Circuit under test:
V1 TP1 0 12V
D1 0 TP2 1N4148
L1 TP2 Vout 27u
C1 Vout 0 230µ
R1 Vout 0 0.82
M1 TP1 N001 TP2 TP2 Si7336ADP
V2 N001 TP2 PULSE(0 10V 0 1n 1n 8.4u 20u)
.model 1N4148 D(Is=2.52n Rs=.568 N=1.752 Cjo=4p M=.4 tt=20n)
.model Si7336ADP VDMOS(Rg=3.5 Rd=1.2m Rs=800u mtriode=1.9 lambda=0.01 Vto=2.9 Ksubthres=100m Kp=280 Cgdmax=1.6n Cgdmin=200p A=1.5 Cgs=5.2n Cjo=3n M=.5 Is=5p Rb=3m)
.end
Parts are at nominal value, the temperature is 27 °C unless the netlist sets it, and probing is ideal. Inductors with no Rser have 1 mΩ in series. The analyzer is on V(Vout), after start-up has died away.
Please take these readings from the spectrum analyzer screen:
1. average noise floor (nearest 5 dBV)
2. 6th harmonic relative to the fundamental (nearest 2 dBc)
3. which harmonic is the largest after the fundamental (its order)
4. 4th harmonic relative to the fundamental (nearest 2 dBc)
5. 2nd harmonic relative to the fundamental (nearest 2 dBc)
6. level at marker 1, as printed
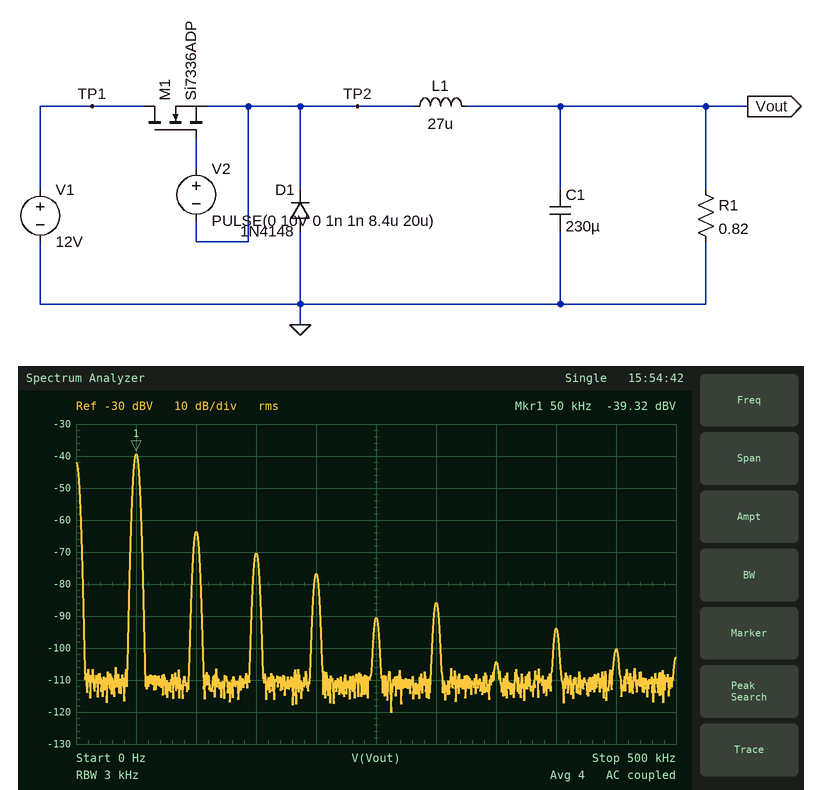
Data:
-110 dBV
-46 dBc
2
-38 dBc
-24 dBc
-39.32 dBV
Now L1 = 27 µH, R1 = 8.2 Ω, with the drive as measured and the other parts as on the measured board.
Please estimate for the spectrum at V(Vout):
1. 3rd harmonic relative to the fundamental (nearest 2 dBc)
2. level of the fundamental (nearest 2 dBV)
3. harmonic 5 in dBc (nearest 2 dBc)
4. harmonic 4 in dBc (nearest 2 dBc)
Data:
-36 dBc
-42 dBV
-44 dBc
-36 dBc
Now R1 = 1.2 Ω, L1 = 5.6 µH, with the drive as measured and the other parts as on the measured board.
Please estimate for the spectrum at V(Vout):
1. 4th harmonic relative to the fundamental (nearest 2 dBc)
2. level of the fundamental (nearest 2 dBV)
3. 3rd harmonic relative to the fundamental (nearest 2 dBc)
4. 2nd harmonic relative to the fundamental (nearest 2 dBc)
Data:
-36 dBc
-26 dBV
-34 dBc
-22 dBc
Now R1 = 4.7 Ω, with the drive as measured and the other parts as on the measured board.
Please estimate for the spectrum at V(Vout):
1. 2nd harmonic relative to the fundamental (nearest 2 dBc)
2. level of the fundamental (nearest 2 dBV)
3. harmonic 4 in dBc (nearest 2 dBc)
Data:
-30 dBc
-40 dBV
-42 dBc
